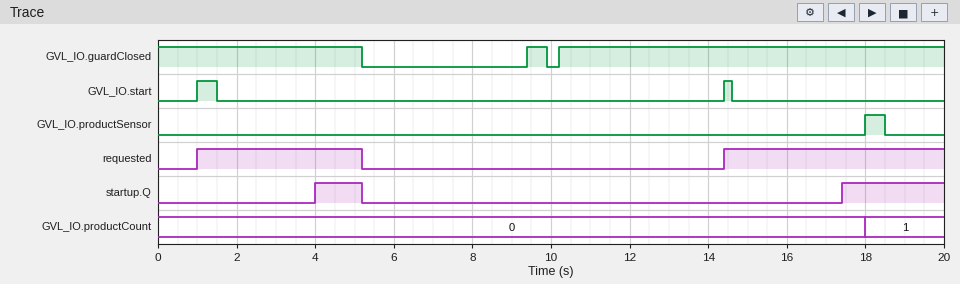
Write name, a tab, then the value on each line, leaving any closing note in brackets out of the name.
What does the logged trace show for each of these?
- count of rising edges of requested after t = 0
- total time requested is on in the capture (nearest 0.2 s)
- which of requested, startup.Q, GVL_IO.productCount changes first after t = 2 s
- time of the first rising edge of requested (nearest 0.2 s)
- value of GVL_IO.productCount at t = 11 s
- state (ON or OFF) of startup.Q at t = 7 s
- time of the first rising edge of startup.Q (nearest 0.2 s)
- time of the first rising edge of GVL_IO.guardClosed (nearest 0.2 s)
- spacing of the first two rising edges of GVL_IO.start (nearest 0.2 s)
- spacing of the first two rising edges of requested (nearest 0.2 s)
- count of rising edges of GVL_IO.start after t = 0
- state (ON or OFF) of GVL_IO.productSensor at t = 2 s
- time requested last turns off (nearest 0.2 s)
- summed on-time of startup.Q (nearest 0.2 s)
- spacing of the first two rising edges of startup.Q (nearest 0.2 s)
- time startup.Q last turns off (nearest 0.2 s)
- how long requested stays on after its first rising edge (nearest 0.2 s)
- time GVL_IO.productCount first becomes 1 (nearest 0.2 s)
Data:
count of rising edges of requested after t = 0	2
total time requested is on in the capture	9.8 s
which of requested, startup.Q, GVL_IO.productCount changes first after t = 2 s	startup.Q
time of the first rising edge of requested	1.0 s
value of GVL_IO.productCount at t = 11 s	0
state (ON or OFF) of startup.Q at t = 7 s	OFF
time of the first rising edge of startup.Q	4.0 s
time of the first rising edge of GVL_IO.guardClosed	9.4 s
spacing of the first two rising edges of GVL_IO.start	13.4 s
spacing of the first two rising edges of requested	13.4 s
count of rising edges of GVL_IO.start after t = 0	2
state (ON or OFF) of GVL_IO.productSensor at t = 2 s	OFF
time requested last turns off	5.2 s
summed on-time of startup.Q	3.8 s
spacing of the first two rising edges of startup.Q	13.4 s
time startup.Q last turns off	5.2 s
how long requested stays on after its first rising edge	4.2 s
time GVL_IO.productCount first becomes 1	18.0 s
